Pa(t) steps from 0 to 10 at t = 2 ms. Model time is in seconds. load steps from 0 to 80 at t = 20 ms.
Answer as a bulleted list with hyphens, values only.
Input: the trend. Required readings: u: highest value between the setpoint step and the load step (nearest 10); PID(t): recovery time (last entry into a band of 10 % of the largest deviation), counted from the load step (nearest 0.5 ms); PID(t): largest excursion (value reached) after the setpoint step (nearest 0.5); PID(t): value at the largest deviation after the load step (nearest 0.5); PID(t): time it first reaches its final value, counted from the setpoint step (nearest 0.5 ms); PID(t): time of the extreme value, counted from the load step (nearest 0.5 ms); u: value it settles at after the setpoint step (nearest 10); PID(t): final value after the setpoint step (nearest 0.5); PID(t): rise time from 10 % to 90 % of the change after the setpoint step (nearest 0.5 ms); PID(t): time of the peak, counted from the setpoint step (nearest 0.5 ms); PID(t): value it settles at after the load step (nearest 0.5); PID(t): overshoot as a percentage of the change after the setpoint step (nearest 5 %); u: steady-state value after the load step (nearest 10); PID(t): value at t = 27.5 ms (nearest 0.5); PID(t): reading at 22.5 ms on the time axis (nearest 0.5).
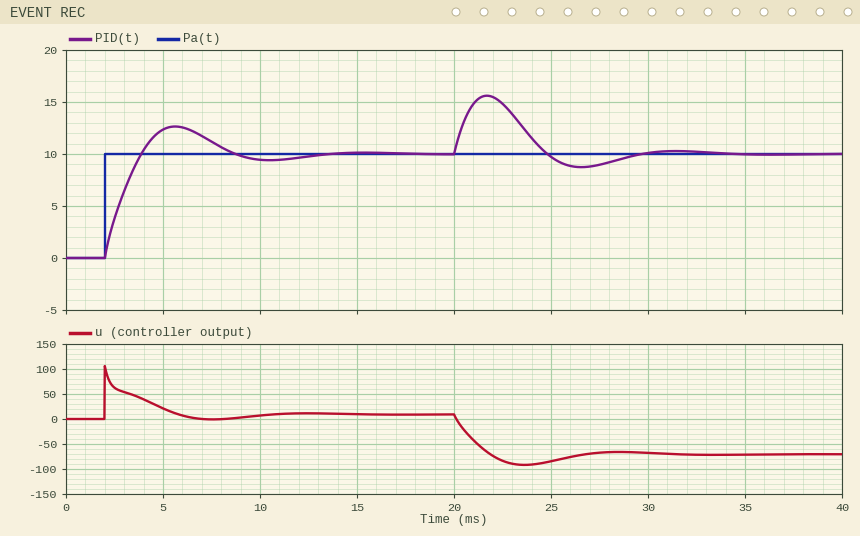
- 110
- 8.5 ms
- 12.5
- 15.5
- 2.0 ms
- 1.5 ms
- 10
- 10.0
- 1.5 ms
- 3.5 ms
- 10.0
- 25 %
- -70
- 9.0
- 15.0
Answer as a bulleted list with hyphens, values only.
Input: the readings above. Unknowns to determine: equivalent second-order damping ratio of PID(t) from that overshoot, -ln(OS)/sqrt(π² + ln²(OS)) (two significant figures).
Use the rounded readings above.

- 0.40
